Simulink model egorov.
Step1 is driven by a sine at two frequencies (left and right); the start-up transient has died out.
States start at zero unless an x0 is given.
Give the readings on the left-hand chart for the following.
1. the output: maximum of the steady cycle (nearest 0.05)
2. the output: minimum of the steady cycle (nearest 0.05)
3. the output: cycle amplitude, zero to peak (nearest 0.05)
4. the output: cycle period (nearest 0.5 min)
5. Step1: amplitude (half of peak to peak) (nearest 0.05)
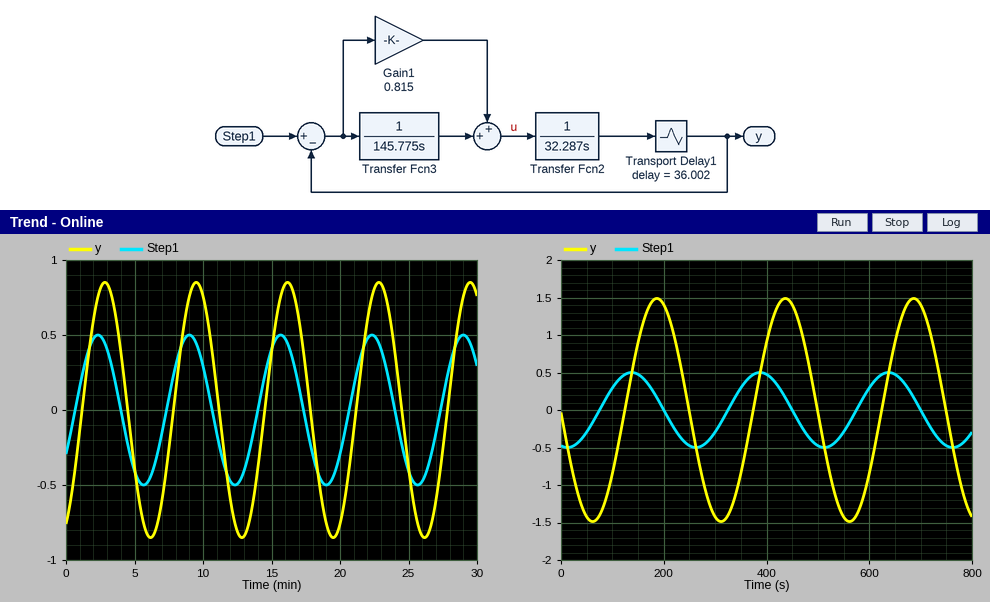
0.85
-0.85
0.85
6.5 min
0.50
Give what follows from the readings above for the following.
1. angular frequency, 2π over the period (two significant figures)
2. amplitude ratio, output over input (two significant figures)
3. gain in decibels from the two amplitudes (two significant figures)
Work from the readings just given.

0.97 rad/min
1.7
4.6 dB
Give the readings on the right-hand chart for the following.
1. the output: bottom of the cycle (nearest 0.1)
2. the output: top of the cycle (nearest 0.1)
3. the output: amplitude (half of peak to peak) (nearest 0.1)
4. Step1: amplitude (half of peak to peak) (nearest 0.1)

-1.5
1.5
1.5
0.5
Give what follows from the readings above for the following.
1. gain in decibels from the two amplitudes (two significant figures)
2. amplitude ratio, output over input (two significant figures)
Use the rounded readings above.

9.5 dB
3.0
